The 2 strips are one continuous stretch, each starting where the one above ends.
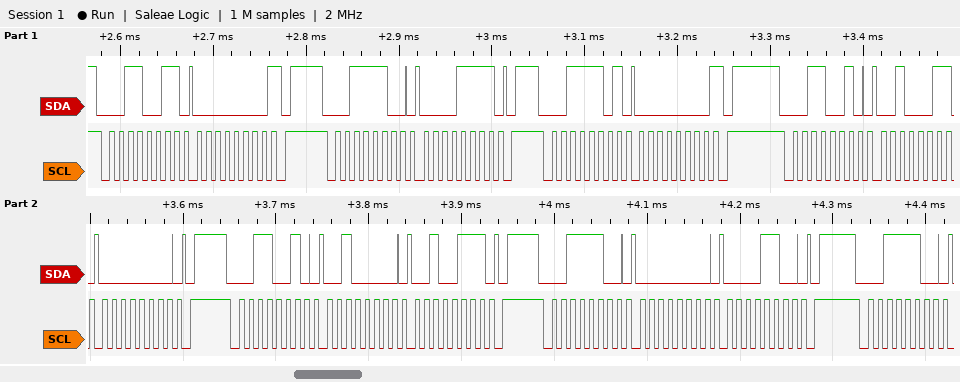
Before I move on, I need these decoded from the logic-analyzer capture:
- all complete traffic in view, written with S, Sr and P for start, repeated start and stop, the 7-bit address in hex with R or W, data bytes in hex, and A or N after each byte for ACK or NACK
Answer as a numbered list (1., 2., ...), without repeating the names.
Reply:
1. S 19R A 00 N P S 1EW A 0F A P S 1ER A 00 N P S 19W A 23 A 00 A P S 19W A 20 A 27 A P S 1EW A 00 A 0C A P S 1EW A
